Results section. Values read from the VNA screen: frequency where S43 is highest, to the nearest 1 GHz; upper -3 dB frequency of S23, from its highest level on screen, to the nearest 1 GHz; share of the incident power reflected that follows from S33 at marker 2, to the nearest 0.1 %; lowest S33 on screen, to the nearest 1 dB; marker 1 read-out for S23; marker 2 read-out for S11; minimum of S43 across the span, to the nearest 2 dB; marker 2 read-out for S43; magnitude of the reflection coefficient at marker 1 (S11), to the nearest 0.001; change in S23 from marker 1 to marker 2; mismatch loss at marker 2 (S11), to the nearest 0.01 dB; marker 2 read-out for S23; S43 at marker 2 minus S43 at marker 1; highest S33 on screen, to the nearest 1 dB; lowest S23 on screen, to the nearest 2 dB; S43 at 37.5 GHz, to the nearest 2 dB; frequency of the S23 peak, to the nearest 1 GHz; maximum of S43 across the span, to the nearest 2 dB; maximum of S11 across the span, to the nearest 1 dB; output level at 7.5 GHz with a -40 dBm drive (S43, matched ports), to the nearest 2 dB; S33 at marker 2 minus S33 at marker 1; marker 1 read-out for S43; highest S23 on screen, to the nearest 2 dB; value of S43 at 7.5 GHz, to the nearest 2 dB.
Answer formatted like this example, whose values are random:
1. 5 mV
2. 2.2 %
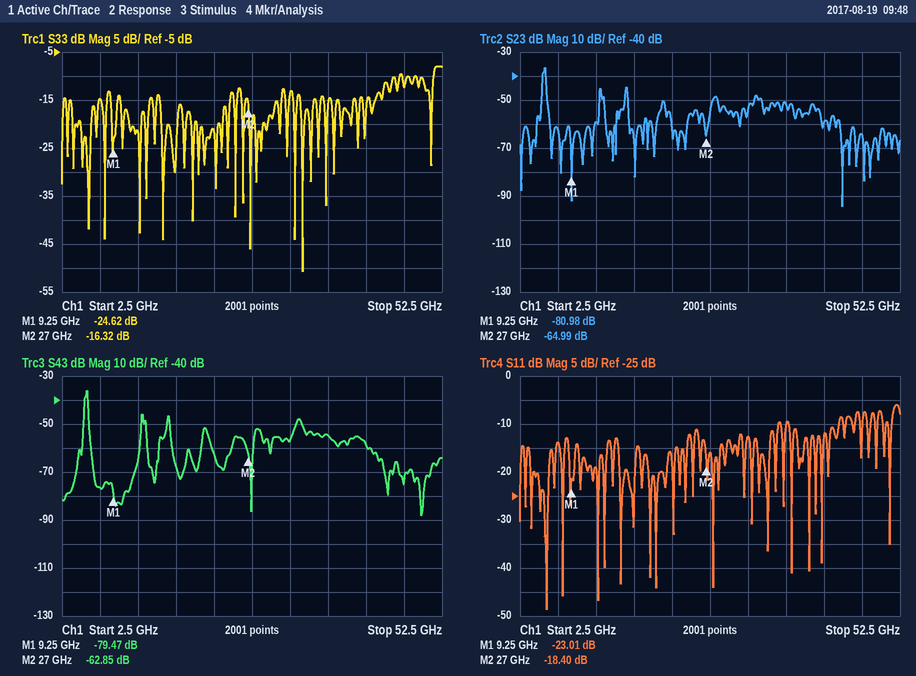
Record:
1. 6 GHz
2. 6 GHz
3. 2.3 %
4. -51 dB
5. -80.98 dB
6. -18.40 dB
7. -88 dB
8. -62.85 dB
9. 0.071
10. 15.99 dB
11. 0.06 dB
12. -64.99 dB
13. 16.62 dB
14. -8 dB
15. -94 dB
16. -54 dB
17. 6 GHz
18. -36 dB
19. -6 dB
20. -116 dBm
21. 8.30 dB
22. -79.47 dB
23. -36 dB
24. -76 dB
